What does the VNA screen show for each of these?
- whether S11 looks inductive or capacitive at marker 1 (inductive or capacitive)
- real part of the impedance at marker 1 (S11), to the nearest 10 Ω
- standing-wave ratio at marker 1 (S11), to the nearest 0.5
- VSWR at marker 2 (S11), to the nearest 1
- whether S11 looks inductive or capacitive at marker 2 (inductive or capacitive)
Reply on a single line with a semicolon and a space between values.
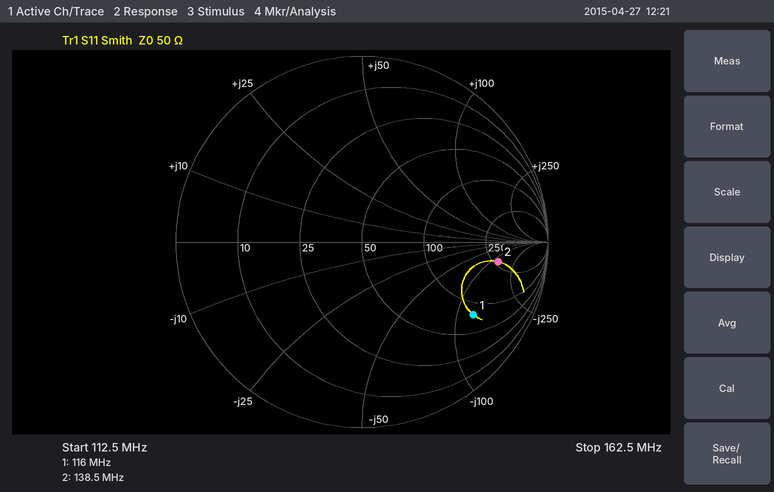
capacitive; 80 Ω; 6.0; 7; capacitive
